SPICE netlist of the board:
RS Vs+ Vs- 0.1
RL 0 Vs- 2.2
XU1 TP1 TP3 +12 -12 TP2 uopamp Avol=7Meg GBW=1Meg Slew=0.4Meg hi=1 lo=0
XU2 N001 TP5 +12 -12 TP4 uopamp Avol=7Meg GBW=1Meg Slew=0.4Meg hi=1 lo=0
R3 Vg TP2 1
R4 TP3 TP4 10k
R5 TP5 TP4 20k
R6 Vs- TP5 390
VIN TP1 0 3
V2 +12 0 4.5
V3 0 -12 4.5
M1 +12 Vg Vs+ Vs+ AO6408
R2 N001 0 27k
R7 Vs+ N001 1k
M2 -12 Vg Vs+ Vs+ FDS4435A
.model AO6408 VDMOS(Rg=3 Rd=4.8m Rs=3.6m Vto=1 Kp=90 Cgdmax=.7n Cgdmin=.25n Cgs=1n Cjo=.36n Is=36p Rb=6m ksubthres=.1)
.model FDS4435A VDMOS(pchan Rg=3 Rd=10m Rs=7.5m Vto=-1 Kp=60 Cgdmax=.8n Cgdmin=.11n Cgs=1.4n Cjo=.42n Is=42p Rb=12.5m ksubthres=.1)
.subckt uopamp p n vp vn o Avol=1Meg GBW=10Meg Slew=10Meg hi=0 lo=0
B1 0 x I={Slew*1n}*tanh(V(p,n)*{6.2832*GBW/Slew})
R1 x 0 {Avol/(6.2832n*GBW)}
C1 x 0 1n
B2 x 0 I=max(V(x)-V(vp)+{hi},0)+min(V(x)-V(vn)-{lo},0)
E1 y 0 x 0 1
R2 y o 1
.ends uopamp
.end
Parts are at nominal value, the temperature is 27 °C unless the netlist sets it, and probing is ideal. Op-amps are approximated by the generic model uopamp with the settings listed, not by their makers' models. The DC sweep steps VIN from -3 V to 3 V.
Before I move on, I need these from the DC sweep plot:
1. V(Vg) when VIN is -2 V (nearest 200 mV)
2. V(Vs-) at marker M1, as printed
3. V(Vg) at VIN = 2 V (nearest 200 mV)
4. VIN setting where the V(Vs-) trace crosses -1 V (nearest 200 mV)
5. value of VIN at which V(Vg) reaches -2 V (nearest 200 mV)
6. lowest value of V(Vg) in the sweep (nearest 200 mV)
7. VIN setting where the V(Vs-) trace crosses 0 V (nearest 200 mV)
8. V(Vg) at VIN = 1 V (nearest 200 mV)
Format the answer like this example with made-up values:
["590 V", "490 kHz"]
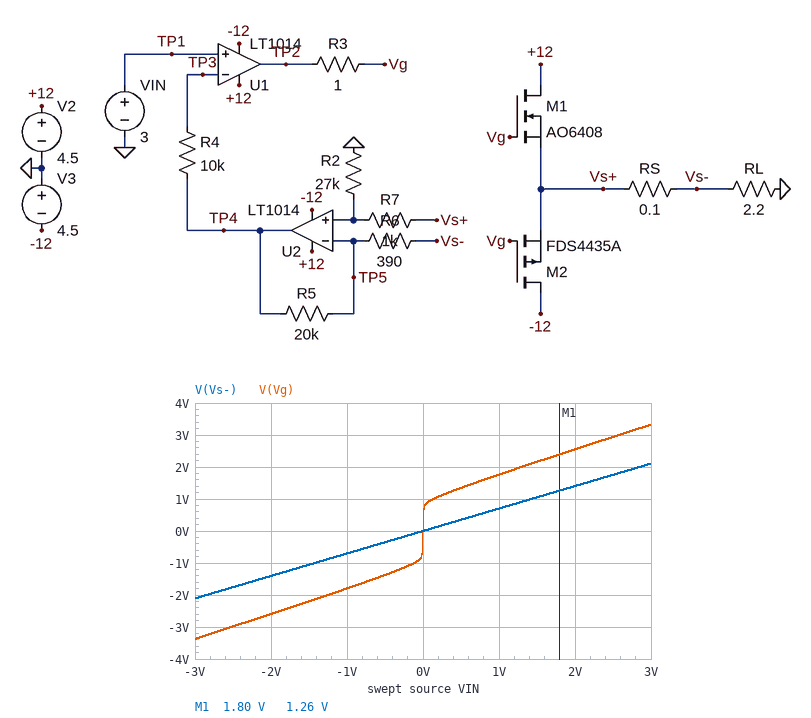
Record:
["-2.6 V", "1.26 V", "2.6 V", "-1.4 V", "-1.2 V", "-3.4 V", "0 V", "1.8 V"]
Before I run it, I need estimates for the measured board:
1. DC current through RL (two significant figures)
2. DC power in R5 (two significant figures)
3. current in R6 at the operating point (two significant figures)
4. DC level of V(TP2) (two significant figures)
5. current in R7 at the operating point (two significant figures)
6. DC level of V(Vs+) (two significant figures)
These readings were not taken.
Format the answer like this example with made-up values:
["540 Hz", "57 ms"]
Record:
["960 mA", "38 µW", "44 µA", "3.3 V", "79 µA", "2.2 V"]
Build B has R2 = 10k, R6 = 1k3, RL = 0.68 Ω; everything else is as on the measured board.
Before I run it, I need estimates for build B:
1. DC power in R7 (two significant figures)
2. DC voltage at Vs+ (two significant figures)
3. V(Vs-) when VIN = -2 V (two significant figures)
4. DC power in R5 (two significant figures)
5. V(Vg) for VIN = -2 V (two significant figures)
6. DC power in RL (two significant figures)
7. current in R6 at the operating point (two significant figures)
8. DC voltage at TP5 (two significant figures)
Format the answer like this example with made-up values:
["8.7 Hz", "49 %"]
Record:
["34 µW", "2.0 V", "-1.2 V", "67 µW", "-2.6 V", "4.6 W", "58 µA", "1.8 V"]
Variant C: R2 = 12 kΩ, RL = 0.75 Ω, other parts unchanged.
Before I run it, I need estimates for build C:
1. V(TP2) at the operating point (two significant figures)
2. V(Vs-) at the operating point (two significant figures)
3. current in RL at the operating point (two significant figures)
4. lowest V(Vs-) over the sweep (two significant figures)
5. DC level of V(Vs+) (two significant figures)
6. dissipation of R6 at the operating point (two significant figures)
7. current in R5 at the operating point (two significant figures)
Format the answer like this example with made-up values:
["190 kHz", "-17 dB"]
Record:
["2.1 V", "880 mV", "1.2 A", "-880 mV", "1.0 V", "4.2 µW", "100 µA"]
